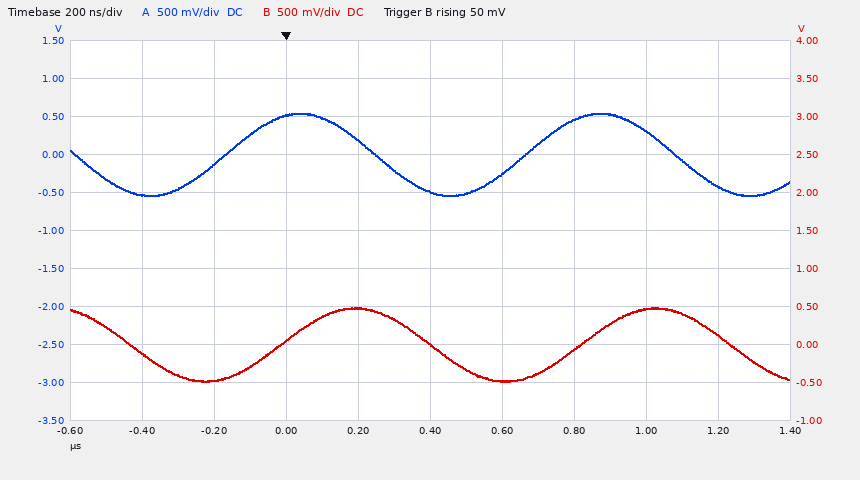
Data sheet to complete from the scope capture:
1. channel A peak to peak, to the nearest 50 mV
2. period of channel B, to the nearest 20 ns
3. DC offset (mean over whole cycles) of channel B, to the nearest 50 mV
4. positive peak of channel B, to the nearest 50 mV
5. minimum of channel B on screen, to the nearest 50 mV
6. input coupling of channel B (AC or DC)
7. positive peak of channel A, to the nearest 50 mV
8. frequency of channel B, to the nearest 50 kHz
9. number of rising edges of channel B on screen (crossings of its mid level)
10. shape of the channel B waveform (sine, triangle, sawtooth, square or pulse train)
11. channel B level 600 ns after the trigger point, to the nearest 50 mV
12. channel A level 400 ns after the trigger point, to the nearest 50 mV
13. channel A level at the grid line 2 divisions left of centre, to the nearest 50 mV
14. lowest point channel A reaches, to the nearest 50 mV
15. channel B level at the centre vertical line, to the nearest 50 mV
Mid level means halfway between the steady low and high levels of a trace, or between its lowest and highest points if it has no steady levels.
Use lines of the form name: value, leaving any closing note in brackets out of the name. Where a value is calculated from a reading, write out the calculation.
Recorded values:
channel A peak to peak, to the nearest 50 mV: 550 mV − (-550 mV) = 1.10 V
period of channel B, to the nearest 20 ns: 840 ns
DC offset (mean over whole cycles) of channel B, to the nearest 50 mV: (500 mV + (-500 mV)) / 2 ≈ 0 mV
positive peak of channel B, to the nearest 50 mV: 500 mV
minimum of channel B on screen, to the nearest 50 mV: -500 mV
input coupling of channel B: DC
positive peak of channel A, to the nearest 50 mV: 550 mV
frequency of channel B, to the nearest 50 kHz: 1 / 840 ns ≈ 1.19 MHz, so 1.20 MHz to the nearest 50 kHz
number of rising edges of channel B on screen: 2
shape of the channel B waveform: sine
channel B level 600 ns after the trigger point, to the nearest 50 mV: -500 mV
channel A level 400 ns after the trigger point, to the nearest 50 mV: -500 mV
channel A level at the grid line 2 divisions left of centre, to the nearest 50 mV: 500 mV
lowest point channel A reaches, to the nearest 50 mV: -550 mV
channel B level at the centre vertical line, to the nearest 50 mV: 0 mV
